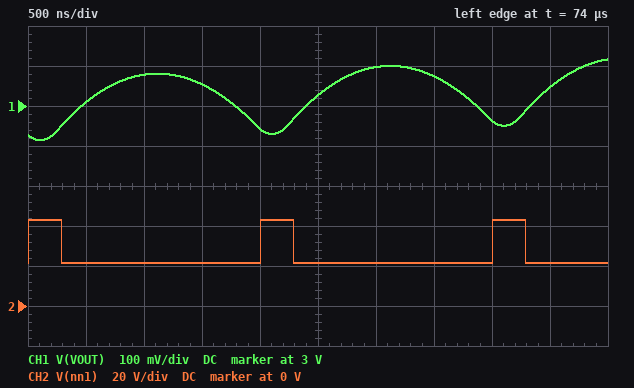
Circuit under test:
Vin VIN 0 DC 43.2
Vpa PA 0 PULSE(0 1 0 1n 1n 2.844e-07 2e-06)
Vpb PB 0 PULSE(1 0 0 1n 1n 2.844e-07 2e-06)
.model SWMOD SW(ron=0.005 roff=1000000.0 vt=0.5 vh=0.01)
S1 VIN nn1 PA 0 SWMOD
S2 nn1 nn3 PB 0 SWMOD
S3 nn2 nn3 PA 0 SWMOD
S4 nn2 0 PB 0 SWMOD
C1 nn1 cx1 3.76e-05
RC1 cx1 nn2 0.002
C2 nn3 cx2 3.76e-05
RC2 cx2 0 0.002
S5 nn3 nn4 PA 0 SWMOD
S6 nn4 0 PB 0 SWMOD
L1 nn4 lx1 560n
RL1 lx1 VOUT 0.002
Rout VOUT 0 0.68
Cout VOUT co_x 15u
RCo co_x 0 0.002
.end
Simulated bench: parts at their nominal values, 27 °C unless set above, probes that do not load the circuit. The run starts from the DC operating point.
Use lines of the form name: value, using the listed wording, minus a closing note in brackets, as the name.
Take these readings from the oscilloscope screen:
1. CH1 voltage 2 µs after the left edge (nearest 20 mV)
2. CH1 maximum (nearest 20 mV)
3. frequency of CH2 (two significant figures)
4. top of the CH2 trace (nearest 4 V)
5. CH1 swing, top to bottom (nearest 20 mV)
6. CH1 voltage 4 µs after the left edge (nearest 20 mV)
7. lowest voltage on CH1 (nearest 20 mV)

CH1 voltage 2 µs after the left edge: 2.94 V
CH1 maximum: 3.12 V
frequency of CH2: 500 kHz
top of the CH2 trace: 44 V
CH1 swing, top to bottom: 200 mV
CH1 voltage 4 µs after the left edge: 2.96 V
lowest voltage on CH1: 2.92 V
